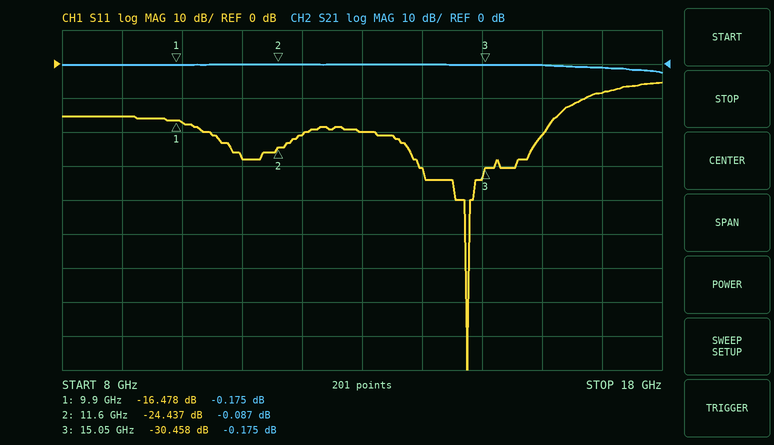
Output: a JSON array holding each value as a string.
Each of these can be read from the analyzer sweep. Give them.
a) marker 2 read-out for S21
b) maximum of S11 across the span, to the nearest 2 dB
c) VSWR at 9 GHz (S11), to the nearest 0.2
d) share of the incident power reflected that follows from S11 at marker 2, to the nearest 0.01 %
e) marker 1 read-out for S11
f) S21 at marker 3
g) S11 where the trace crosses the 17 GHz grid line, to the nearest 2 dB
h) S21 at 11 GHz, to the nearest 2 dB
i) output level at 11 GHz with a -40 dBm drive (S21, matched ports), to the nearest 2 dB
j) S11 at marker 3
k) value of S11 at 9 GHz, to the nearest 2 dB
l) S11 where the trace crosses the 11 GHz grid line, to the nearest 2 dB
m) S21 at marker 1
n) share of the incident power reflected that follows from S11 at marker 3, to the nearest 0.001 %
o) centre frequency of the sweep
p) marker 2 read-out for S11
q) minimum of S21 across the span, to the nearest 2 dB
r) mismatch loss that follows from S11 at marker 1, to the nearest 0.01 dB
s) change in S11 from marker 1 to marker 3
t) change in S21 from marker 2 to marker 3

["-0.087 dB", "-6 dB", "1.4", "0.36 %", "-16.478 dB", "-0.175 dB", "-8 dB", "0 dB", "-40 dBm", "-30.458 dB", "-16 dB", "-28 dB", "-0.175 dB", "0.090 %", "13 GHz", "-24.437 dB", "-2 dB", "0.10 dB", "-13.980 dB", "-0.088 dB"]
